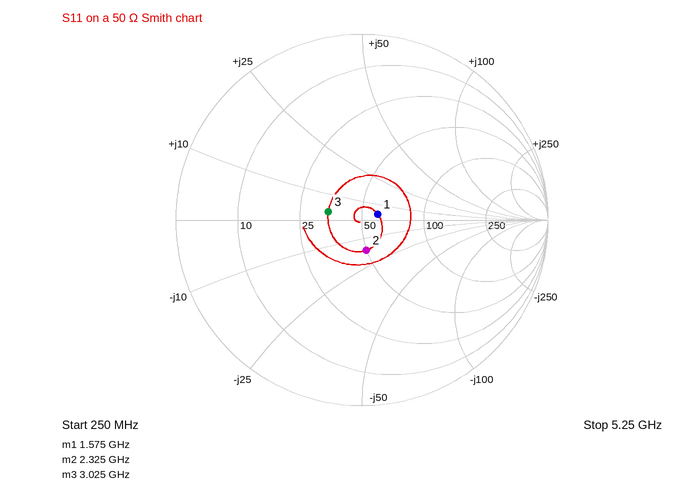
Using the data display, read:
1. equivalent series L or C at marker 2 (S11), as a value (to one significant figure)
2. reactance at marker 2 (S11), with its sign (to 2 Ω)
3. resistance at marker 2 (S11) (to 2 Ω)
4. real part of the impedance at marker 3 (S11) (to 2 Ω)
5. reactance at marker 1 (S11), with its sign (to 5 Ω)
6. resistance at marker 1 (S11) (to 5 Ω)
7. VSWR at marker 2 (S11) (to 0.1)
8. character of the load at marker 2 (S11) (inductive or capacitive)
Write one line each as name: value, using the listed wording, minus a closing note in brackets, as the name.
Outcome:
equivalent series L or C at marker 2 (S11), as a value: 4 pF
reactance at marker 2 (S11), with its sign: -16 Ω
resistance at marker 2 (S11): 50 Ω
real part of the impedance at marker 3 (S11): 34 Ω
reactance at marker 1 (S11), with its sign: +5 Ω
resistance at marker 1 (S11): 60 Ω
VSWR at marker 2 (S11): 1.4
character of the load at marker 2 (S11): capacitive
